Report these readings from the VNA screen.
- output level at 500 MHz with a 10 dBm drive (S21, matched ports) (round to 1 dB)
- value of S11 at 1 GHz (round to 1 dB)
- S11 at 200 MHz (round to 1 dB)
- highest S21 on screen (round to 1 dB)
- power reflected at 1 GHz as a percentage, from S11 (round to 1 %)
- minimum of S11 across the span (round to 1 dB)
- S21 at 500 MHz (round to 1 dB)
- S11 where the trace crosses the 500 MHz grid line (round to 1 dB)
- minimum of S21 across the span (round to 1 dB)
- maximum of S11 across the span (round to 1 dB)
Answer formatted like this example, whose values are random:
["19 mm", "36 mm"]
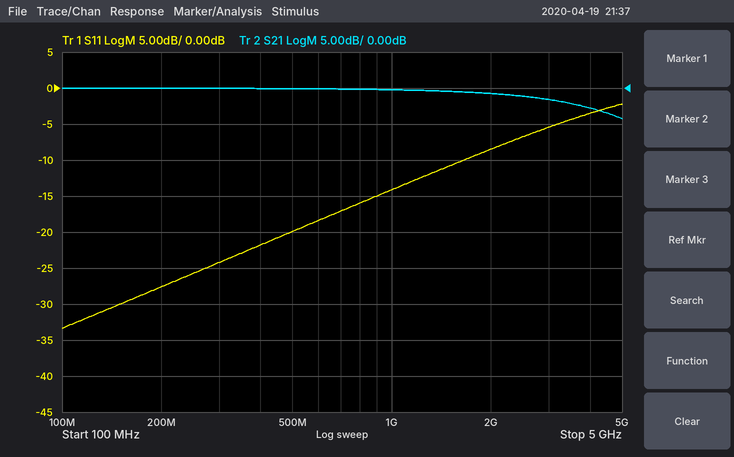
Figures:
["10 dBm", "-14 dB", "-28 dB", "0 dB", "4 %", "-33 dB", "0 dB", "-20 dB", "-4 dB", "-2 dB"]
